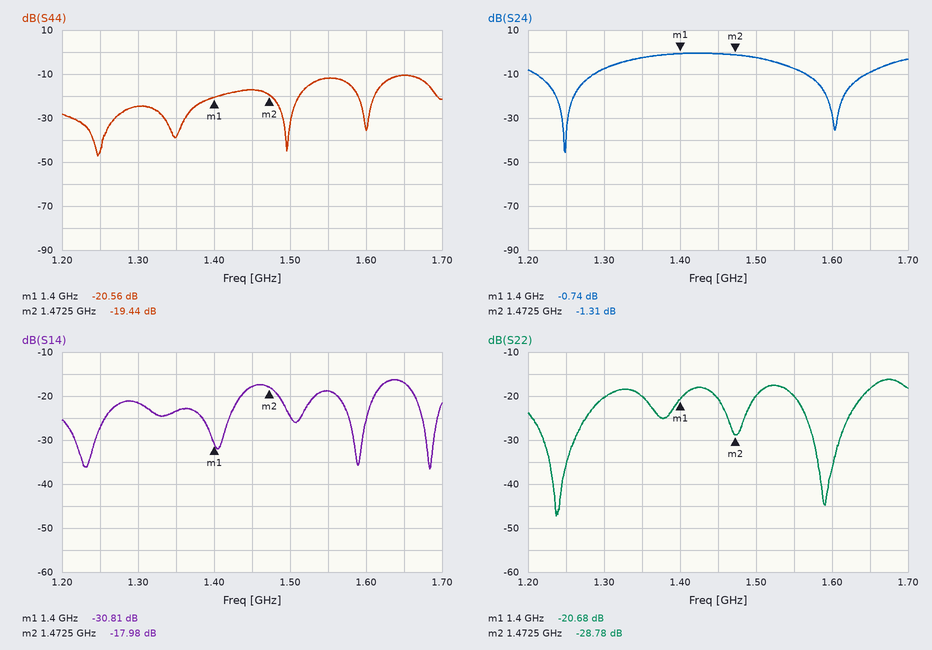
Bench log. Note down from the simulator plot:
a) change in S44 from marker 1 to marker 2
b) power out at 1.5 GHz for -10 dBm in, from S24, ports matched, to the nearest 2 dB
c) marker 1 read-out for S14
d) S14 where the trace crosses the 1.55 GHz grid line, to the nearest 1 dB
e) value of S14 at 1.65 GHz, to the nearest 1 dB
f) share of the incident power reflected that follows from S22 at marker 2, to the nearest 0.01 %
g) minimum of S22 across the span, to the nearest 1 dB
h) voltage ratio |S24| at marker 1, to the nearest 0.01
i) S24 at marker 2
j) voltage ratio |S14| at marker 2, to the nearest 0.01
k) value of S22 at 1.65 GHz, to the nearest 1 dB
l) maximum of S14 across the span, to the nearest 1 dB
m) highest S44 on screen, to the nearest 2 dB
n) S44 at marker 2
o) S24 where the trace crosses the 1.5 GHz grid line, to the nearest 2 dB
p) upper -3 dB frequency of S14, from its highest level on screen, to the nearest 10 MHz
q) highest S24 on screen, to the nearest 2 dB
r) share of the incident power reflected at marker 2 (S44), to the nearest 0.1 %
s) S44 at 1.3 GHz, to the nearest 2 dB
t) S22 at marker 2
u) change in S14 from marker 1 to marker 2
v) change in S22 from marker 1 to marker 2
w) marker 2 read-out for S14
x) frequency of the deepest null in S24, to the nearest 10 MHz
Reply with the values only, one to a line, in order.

1.12 dB
-12 dBm
-30.81 dB
-19 dB
-17 dB
0.13 %
-47 dB
0.92
-1.31 dB
0.13
-18 dB
-16 dB
-10 dB
-19.44 dB
-2 dB
1.66 GHz
0 dB
1.1 %
-24 dB
-28.78 dB
12.83 dB
-8.10 dB
-17.98 dB
1.25 GHz
